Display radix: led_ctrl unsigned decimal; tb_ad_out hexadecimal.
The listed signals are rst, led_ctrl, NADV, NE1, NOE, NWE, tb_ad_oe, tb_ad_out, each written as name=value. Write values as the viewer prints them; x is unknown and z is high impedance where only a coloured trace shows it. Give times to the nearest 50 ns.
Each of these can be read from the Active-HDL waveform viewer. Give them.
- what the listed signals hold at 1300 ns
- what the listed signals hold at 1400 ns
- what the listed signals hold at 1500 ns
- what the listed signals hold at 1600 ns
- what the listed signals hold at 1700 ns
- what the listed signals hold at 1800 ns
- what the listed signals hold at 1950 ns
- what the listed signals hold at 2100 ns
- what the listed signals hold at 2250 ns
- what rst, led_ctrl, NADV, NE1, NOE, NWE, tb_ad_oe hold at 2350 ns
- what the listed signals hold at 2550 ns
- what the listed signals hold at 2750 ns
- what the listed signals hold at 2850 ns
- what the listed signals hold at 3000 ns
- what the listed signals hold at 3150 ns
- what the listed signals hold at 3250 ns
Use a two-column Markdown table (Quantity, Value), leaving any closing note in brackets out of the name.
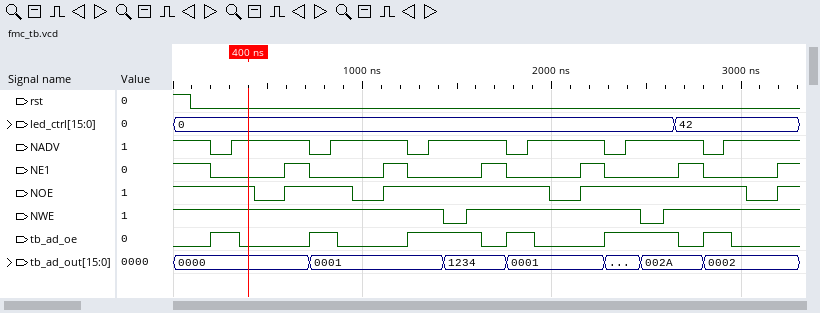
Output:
| Quantity | Value |
|---|---|
| what the listed signals hold at 1300 ns | rst=0, led_ctrl=0, NADV=0, NE1=0, NOE=1, NWE=1, tb_ad_oe=1, tb_ad_out=0001 |
| what the listed signals hold at 1400 ns | rst=0, led_ctrl=0, NADV=1, NE1=0, NOE=1, NWE=1, tb_ad_oe=1, tb_ad_out=0001 |
| what the listed signals hold at 1500 ns | rst=0, led_ctrl=0, NADV=1, NE1=0, NOE=1, NWE=0, tb_ad_oe=1, tb_ad_out=1234 |
| what the listed signals hold at 1600 ns | rst=0, led_ctrl=0, NADV=1, NE1=0, NOE=1, NWE=1, tb_ad_oe=1, tb_ad_out=1234 |
| what the listed signals hold at 1700 ns | rst=0, led_ctrl=0, NADV=1, NE1=1, NOE=1, NWE=1, tb_ad_oe=0, tb_ad_out=1234 |
| what the listed signals hold at 1800 ns | rst=0, led_ctrl=0, NADV=0, NE1=0, NOE=1, NWE=1, tb_ad_oe=1, tb_ad_out=0001 |
| what the listed signals hold at 1950 ns | rst=0, led_ctrl=0, NADV=1, NE1=0, NOE=1, NWE=1, tb_ad_oe=0, tb_ad_out=0001 |
| what the listed signals hold at 2100 ns | rst=0, led_ctrl=0, NADV=1, NE1=0, NOE=0, NWE=1, tb_ad_oe=0, tb_ad_out=0001 |
| what the listed signals hold at 2250 ns | rst=0, led_ctrl=0, NADV=1, NE1=1, NOE=1, NWE=1, tb_ad_oe=0, tb_ad_out=0001 |
| what rst, led_ctrl, NADV, NE1, NOE, NWE, tb_ad_oe hold at 2350 ns | rst=0, led_ctrl=0, NADV=0, NE1=0, NOE=1, NWE=1, tb_ad_oe=1 |
| what the listed signals hold at 2550 ns | rst=0, led_ctrl=0, NADV=1, NE1=0, NOE=1, NWE=0, tb_ad_oe=1, tb_ad_out=002A |
| what the listed signals hold at 2750 ns | rst=0, led_ctrl=42, NADV=1, NE1=1, NOE=1, NWE=1, tb_ad_oe=0, tb_ad_out=002A |
| what the listed signals hold at 2850 ns | rst=0, led_ctrl=42, NADV=0, NE1=0, NOE=1, NWE=1, tb_ad_oe=1, tb_ad_out=0002 |
| what the listed signals hold at 3000 ns | rst=0, led_ctrl=42, NADV=1, NE1=0, NOE=1, NWE=1, tb_ad_oe=0, tb_ad_out=0002 |
| what the listed signals hold at 3150 ns | rst=0, led_ctrl=42, NADV=1, NE1=0, NOE=0, NWE=1, tb_ad_oe=0, tb_ad_out=0002 |
| what the listed signals hold at 3250 ns | rst=0, led_ctrl=42, NADV=1, NE1=1, NOE=1, NWE=1, tb_ad_oe=0, tb_ad_out=0002 |
